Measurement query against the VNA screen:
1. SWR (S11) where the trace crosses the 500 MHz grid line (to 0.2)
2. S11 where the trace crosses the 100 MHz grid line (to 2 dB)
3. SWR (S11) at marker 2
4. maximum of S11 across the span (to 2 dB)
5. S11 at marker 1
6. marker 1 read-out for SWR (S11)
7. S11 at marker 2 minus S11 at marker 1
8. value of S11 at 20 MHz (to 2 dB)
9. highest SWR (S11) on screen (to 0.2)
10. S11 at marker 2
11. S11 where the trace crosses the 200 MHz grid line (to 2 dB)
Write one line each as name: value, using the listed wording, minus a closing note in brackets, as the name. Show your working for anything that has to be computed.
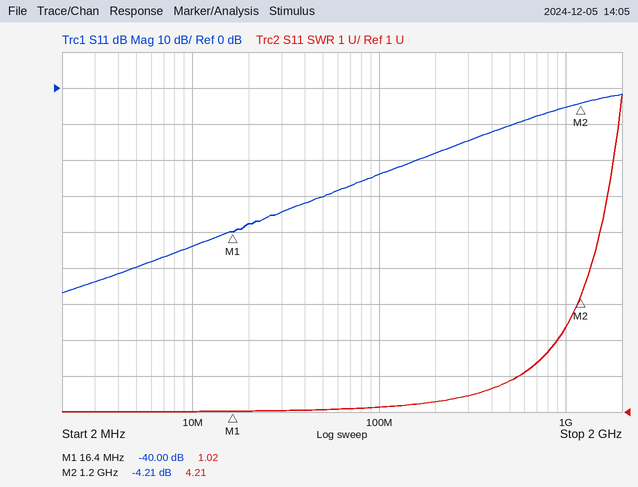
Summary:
SWR (S11) where the trace crosses the 500 MHz grid line: 1.8
S11 where the trace crosses the 100 MHz grid line: -24 dB
SWR (S11) at marker 2: 4.21
maximum of S11 across the span: -2 dB
S11 at marker 1: -40.00 dB
marker 1 read-out for SWR: 1.02
S11 at marker 2 minus S11 at marker 1: -4.21 − (-40) = 35.79 dB
value of S11 at 20 MHz: -38 dB
highest SWR (S11) on screen: 9.8
S11 at marker 2: -4.21 dB
S11 where the trace crosses the 200 MHz grid line: -18 dB
